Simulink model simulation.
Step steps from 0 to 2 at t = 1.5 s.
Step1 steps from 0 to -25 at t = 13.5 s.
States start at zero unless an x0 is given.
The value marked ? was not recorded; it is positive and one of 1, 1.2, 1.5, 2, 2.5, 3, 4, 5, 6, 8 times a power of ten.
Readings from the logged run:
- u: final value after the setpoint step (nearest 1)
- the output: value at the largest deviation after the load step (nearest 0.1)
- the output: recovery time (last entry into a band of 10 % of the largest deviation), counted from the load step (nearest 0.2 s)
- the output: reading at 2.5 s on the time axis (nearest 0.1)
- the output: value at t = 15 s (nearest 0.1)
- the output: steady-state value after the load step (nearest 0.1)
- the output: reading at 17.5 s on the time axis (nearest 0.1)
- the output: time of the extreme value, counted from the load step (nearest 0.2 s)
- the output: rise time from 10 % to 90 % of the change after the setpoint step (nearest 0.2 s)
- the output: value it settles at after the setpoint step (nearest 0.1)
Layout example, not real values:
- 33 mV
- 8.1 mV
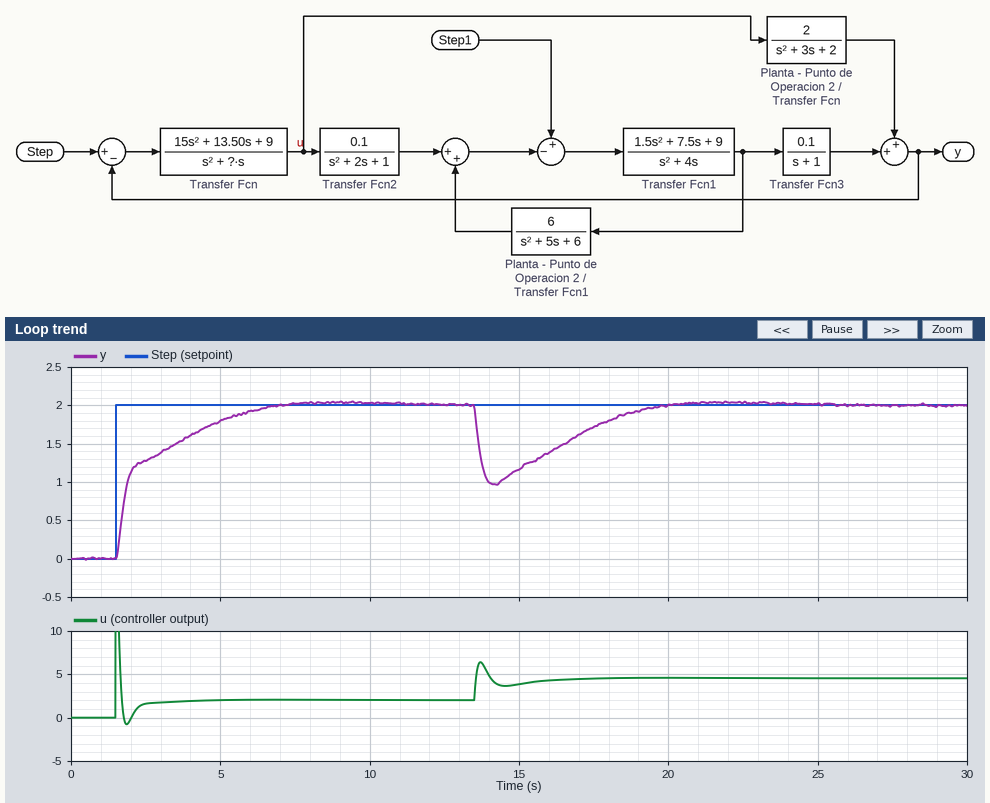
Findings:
- 2
- 1.0
- 5.2 s
- 1.3
- 1.2
- 2.0
- 1.7
- 0.6 s
- 3.4 s
- 2.0
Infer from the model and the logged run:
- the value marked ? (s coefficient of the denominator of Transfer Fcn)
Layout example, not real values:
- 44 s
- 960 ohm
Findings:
- 10
